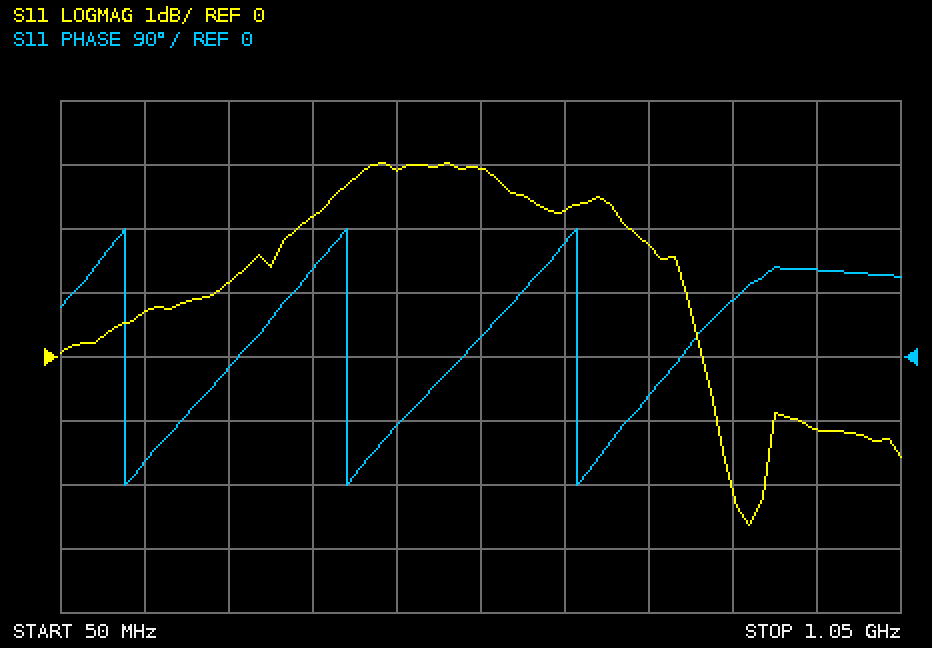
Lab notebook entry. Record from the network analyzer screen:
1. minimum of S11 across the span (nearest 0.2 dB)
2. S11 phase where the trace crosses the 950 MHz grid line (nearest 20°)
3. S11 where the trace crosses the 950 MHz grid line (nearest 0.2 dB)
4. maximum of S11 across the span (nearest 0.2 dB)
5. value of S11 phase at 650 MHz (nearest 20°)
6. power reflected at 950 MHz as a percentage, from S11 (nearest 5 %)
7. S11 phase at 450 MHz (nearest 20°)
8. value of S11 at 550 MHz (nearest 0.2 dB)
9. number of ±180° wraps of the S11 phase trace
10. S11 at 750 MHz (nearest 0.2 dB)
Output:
-2.6 dB
120°
-1.2 dB
3.0 dB
160°
75 %
-100°
3.0 dB
3
1.8 dB
